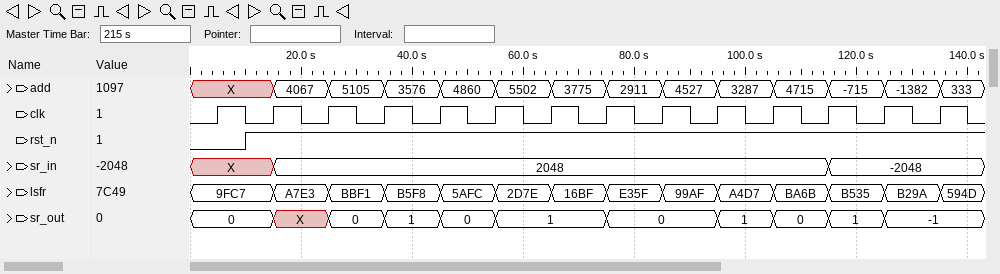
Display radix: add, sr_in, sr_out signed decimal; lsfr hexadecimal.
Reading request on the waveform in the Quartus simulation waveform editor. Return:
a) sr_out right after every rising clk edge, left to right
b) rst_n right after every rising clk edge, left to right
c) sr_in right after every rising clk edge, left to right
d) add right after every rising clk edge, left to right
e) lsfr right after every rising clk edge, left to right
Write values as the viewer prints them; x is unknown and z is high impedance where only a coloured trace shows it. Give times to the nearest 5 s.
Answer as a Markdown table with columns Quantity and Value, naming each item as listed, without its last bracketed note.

| Quantity | Value |
|---|---|
| sr_out right after every rising clk edge, left to right | 0, X, 0, 1, 0, 1, 1, 0, 0, 1, 0, 1, -1, -1 |
| rst_n right after every rising clk edge, left to right | 0 1 1 1 1 1 1 1 1 1 1 1 1 1 |
| sr_in right after every rising clk edge, left to right | X, 2048, 2048, 2048, 2048, 2048, 2048, 2048, 2048, 2048, 2048, -2048, -2048, -2048 |
| add right after every rising clk edge, left to right | X, 4067, 5105, 3576, 4860, 5502, 3775, 2911, 4527, 3287, 4715, -715, -1382, 333 |
| lsfr right after every rising clk edge, left to right | 9FC7, A7E3, BBF1, B5F8, 5AFC, 2D7E, 16BF, E35F, 99AF, A4D7, BA6B, B535, B29A, 594D |
